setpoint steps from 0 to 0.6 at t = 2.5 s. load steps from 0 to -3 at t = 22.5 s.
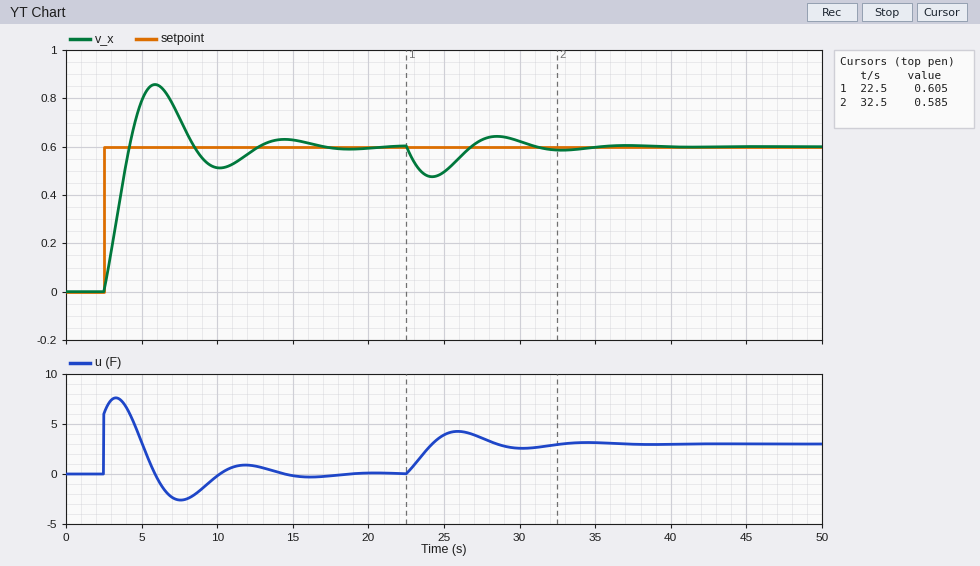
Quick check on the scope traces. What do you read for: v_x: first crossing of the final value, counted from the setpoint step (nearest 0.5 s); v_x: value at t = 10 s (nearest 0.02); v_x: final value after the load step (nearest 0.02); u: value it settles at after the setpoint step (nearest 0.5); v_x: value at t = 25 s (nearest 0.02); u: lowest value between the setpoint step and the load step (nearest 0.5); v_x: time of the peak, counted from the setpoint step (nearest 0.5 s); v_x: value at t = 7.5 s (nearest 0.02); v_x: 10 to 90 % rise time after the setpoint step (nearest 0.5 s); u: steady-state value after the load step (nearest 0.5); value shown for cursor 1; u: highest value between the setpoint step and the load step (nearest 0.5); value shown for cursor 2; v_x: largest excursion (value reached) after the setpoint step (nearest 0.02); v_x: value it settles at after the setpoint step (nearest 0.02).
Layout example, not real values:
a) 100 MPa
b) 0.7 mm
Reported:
a) 1.5 s
b) 0.52
c) 0.60
d) 0.0
e) 0.50
f) -2.5
g) 3.5 s
h) 0.72
i) 1.5 s
j) 3.0
k) 0.605
l) 7.5
m) 0.585
n) 0.86
o) 0.60
